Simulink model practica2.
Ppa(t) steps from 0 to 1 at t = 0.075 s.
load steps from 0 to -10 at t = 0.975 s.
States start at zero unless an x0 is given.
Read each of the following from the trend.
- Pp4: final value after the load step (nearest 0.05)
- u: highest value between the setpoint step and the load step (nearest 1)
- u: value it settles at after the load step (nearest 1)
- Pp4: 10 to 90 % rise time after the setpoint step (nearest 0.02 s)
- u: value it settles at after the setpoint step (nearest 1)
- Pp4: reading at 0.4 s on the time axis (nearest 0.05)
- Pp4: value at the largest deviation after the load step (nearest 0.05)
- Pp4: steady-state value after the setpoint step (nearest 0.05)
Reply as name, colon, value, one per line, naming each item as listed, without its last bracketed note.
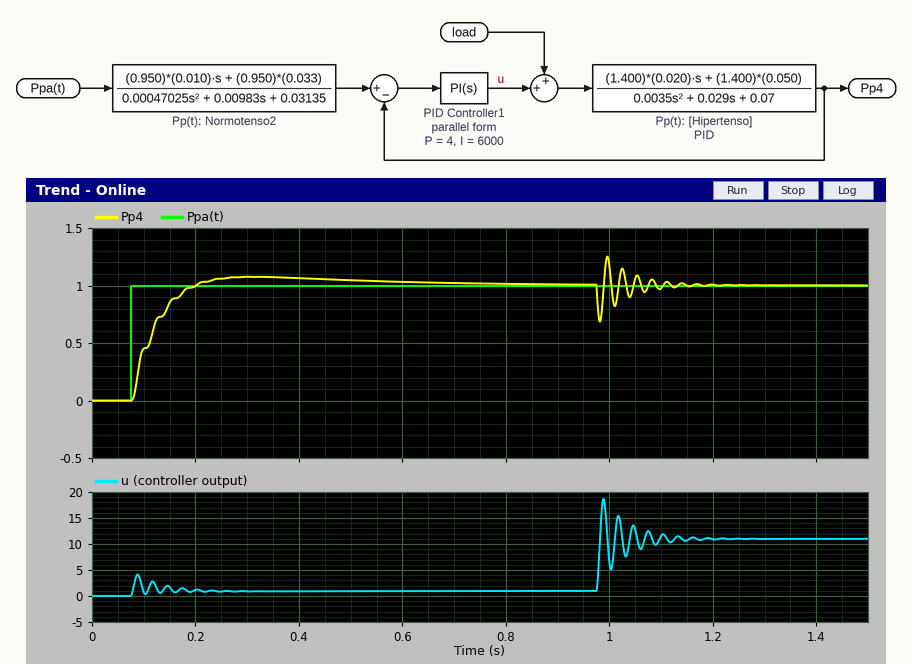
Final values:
Pp4: final value after the load step: 1.00
u: highest value between the setpoint step and the load step: 4
u: value it settles at after the load step: 11
Pp4: 10 to 90 % rise time after the setpoint step: 0.08 s
u: value it settles at after the setpoint step: 1
Pp4: reading at 0.4 s on the time axis: 1.05
Pp4: value at the largest deviation after the load step: 0.70
Pp4: steady-state value after the setpoint step: 1.00
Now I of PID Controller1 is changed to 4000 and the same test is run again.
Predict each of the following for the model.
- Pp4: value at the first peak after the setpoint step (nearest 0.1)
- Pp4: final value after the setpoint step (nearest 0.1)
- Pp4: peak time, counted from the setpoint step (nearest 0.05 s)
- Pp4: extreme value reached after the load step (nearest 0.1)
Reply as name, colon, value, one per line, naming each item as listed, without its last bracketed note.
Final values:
Pp4: value at the first peak after the setpoint step: 1.1
Pp4: final value after the setpoint step: 1.0
Pp4: peak time, counted from the setpoint step: 0.25 s
Pp4: extreme value reached after the load step: 0.6
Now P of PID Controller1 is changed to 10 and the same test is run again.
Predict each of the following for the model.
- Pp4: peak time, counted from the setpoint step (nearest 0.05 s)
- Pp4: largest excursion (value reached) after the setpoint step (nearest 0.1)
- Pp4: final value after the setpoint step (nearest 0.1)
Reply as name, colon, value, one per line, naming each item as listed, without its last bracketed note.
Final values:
Pp4: peak time, counted from the setpoint step: 0.25 s
Pp4: largest excursion (value reached) after the setpoint step: 1.1
Pp4: final value after the setpoint step: 1.0
